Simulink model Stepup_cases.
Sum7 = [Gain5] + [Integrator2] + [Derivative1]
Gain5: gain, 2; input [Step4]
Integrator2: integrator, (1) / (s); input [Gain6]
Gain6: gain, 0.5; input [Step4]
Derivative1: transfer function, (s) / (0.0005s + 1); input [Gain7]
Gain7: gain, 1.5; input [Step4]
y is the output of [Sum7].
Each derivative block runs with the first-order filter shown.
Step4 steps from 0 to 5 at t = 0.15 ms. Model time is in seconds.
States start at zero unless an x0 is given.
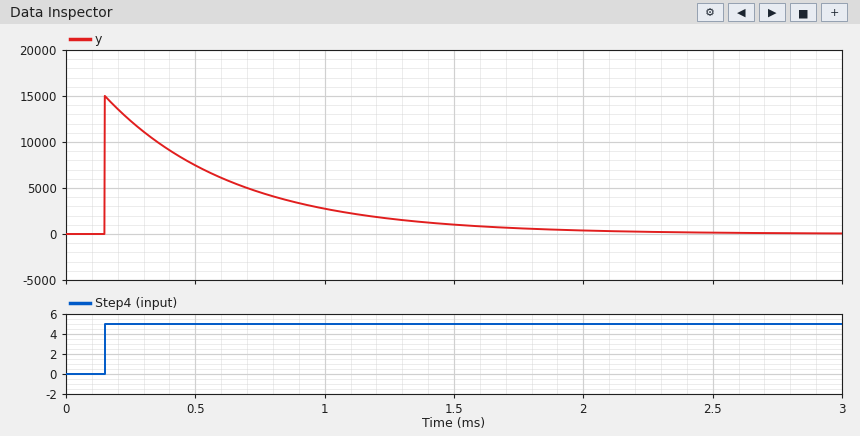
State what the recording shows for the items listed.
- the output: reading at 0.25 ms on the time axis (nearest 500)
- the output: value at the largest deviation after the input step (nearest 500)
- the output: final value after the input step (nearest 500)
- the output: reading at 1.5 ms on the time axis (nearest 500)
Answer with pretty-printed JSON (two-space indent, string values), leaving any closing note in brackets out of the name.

{
  "the output: reading at 0.25 ms on the time axis": "12500",
  "the output: value at the largest deviation after the input step": "15000",
  "the output: final value after the input step": "0",
  "the output: reading at 1.5 ms on the time axis": "1000"
}
